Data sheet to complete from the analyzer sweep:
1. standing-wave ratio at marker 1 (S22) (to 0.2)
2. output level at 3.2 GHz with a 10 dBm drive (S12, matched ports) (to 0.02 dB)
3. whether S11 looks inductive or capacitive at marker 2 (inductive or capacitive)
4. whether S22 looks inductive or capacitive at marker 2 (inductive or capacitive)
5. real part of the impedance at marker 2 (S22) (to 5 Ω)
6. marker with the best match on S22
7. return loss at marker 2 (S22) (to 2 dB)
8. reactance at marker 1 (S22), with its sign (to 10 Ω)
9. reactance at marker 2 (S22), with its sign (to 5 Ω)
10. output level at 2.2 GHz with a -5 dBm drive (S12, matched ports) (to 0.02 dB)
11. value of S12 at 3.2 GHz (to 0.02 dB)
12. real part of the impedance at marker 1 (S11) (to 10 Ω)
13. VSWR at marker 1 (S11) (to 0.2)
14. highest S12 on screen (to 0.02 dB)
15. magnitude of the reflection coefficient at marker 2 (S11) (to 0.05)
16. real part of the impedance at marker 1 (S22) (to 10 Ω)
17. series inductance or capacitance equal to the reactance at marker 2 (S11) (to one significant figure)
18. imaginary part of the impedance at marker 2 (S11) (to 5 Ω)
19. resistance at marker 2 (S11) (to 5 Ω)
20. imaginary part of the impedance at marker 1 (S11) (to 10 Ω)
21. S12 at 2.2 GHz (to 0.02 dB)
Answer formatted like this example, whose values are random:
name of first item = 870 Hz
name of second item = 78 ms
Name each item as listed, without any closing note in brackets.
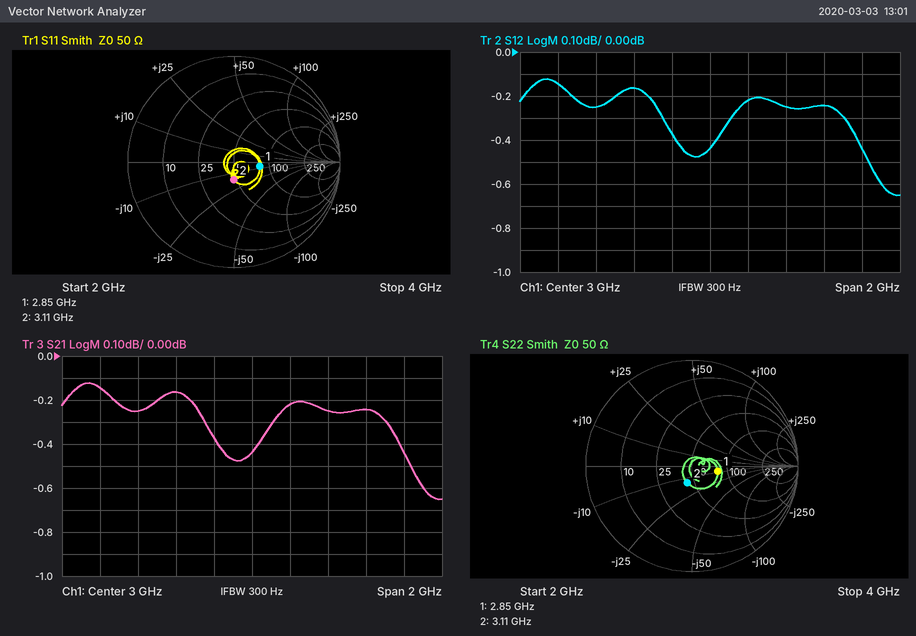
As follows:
standing-wave ratio at marker 1 (S22) = 1.6
output level at 3.2 GHz with a 10 dBm drive (S12, matched ports) = 9.78 dBm
whether S11 looks inductive or capacitive at marker 2 = capacitive
whether S22 looks inductive or capacitive at marker 2 = capacitive
real part of the impedance at marker 2 (S22) = 45 Ω
marker with the best match on S22 = marker 2
return loss at marker 2 (S22) = 16 dB
reactance at marker 1 (S22), with its sign = -10 Ω
reactance at marker 2 (S22), with its sign = -15 Ω
output level at 2.2 GHz with a -5 dBm drive (S12, matched ports) = -5.14 dBm
value of S12 at 3.2 GHz = -0.22 dB
real part of the impedance at marker 1 (S11) = 80 Ω
VSWR at marker 1 (S11) = 1.6
highest S12 on screen = -0.12 dB
magnitude of the reflection coefficient at marker 2 (S11) = 0.15
real part of the impedance at marker 1 (S22) = 80 Ω
series inductance or capacitance equal to the reactance at marker 2 (S11) = 3 pF
imaginary part of the impedance at marker 2 (S11) = -15 Ω
resistance at marker 2 (S11) = 45 Ω
imaginary part of the impedance at marker 1 (S11) = -10 Ω
S12 at 2.2 GHz = -0.14 dB
